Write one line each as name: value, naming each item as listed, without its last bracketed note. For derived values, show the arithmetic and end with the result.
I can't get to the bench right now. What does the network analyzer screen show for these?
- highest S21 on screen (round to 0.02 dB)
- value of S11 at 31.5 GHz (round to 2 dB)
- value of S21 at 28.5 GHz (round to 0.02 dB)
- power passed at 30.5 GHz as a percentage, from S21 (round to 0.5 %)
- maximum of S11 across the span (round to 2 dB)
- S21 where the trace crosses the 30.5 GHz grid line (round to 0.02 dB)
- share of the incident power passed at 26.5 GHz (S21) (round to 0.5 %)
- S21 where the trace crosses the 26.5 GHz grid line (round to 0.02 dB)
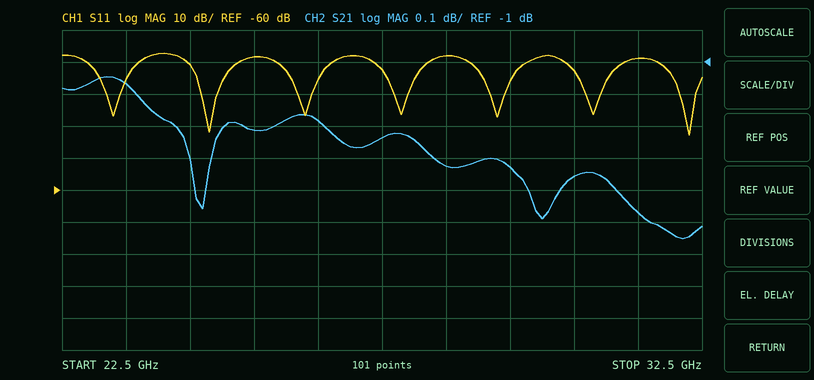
highest S21 on screen: -1.04 dB
value of S11 at 31.5 GHz: -18 dB
value of S21 at 28.5 GHz: -1.32 dB
power passed at 30.5 GHz as a percentage, from S21: 10^(-1.36/10) ≈ 73.1 %, so 73.0 % to the nearest 0.5 %
maximum of S11 across the span: -18 dB
S21 where the trace crosses the 30.5 GHz grid line: -1.36 dB
share of the incident power passed at 26.5 GHz (S21): 10^(-1.18/10) ≈ 76.2 %, so 76.0 % to the nearest 0.5 %
S21 where the trace crosses the 26.5 GHz grid line: -1.18 dB
